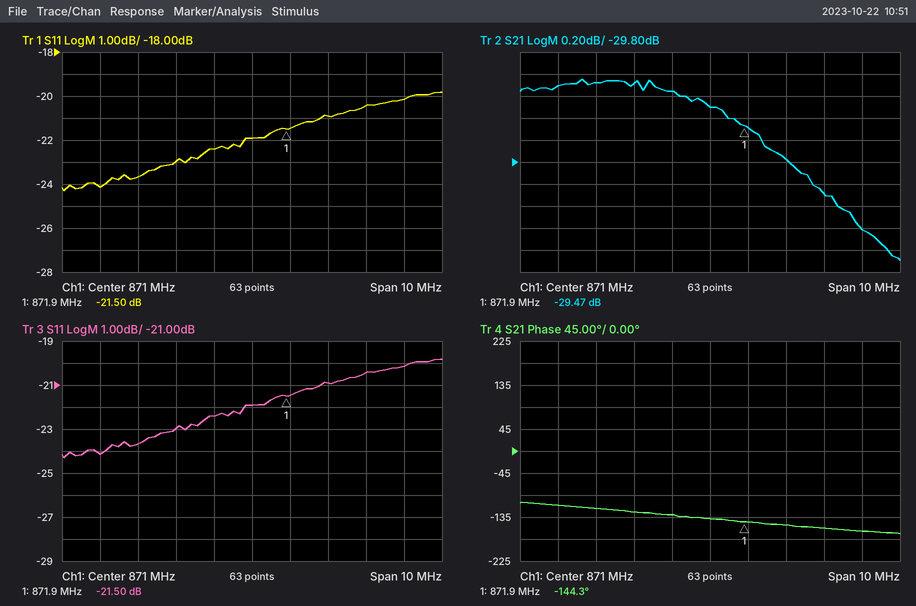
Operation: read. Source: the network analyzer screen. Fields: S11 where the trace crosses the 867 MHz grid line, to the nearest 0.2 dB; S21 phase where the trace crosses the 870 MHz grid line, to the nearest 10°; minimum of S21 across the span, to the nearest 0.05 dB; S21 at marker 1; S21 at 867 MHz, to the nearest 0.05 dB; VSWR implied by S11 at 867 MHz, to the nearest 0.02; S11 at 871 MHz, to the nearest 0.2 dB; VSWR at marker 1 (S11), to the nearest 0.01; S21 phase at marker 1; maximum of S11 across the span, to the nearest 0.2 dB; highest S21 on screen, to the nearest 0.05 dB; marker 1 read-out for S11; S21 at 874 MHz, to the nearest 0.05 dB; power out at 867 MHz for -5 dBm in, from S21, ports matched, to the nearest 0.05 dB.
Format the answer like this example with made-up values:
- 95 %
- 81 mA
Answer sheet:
- -24.2 dB
- -130°
- -30.70 dB
- -29.47 dB
- -29.10 dB
- 1.14
- -22.0 dB
- 1.18
- -144.3°
- -19.8 dB
- -29.05 dB
- -21.50 dB
- -30.10 dB
- -34.10 dBm
